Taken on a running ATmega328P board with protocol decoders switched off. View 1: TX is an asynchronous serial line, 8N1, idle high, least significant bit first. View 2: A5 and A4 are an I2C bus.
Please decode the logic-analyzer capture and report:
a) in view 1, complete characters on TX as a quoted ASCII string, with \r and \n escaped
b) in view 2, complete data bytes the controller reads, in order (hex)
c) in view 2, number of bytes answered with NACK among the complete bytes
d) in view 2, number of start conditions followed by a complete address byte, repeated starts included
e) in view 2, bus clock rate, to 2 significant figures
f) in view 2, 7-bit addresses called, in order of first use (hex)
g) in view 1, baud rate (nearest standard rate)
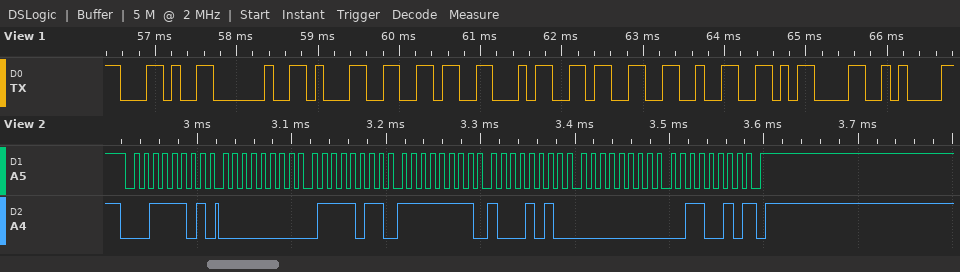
", 16432\r\n"
00 7B FF 8A 00 32
1
1
100 kHz
0x1E
9600 baud
